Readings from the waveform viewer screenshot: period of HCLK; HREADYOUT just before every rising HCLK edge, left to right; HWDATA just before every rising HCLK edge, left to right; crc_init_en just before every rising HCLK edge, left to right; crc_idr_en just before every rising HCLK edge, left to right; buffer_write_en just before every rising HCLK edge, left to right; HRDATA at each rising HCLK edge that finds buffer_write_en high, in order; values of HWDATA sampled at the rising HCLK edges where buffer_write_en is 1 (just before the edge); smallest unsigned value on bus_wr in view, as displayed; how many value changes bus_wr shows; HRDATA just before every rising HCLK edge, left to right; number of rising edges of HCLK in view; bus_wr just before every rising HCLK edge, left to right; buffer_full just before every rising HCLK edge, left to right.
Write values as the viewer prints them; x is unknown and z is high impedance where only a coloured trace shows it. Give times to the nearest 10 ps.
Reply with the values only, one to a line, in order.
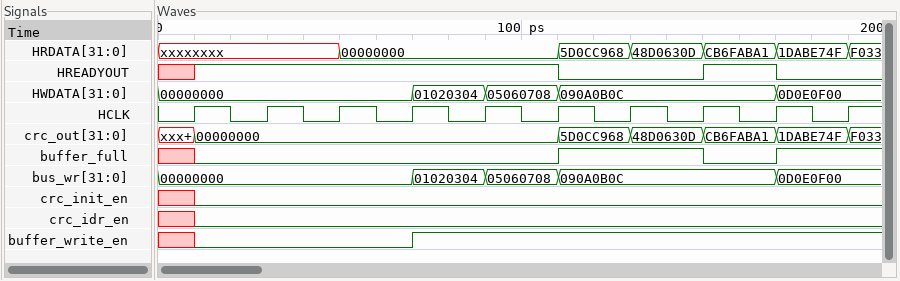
20 ps
x 1 1 1 1 1 0 0 1 0
00000000, 00000000, 00000000, 00000000, 01020304, 05060708, 090A0B0C, 090A0B0C, 090A0B0C, 0D0E0F00
x 0 0 0 0 0 0 0 0 0
x 0 0 0 0 0 0 0 0 0
x 0 0 0 1 1 1 1 1 1
00000000, 00000000, 5D0CC968, 48D0630D, CB6FABA1, 1DABE74F
01020304, 05060708, 090A0B0C, 090A0B0C, 090A0B0C, 0D0E0F00
00000000
4
xxxxxxxx, xxxxxxxx, xxxxxxxx, 00000000, 00000000, 00000000, 5D0CC968, 48D0630D, CB6FABA1, 1DABE74F
10
00000000, 00000000, 00000000, 00000000, 01020304, 05060708, 090A0B0C, 090A0B0C, 090A0B0C, 0D0E0F00
x 0 0 0 0 0 1 1 0 1
